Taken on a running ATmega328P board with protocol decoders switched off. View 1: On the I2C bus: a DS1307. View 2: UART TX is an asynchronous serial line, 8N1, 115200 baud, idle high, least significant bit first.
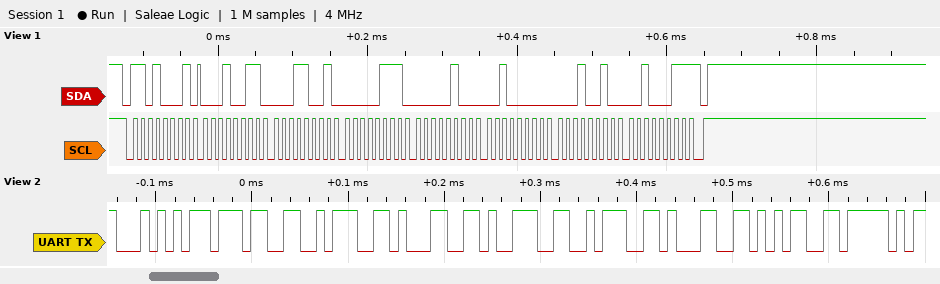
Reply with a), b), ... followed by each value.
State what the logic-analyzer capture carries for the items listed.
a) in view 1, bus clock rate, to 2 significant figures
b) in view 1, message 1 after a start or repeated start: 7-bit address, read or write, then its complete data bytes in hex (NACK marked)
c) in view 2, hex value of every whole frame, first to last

a) 100 kHz
b) 0x68 read: 13 19 07 04 20 12 23 NACK
c) 54 37 3A 31 39 3A 31 35 5F
